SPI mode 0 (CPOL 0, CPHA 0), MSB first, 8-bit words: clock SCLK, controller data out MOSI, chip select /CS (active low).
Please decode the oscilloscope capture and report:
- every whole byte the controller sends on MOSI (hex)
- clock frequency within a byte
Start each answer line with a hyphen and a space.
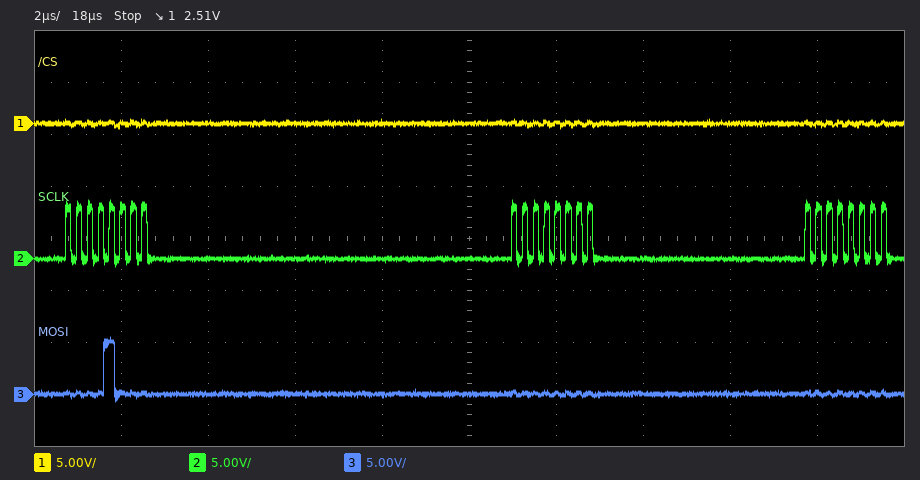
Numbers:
- 08 00 00
- 4 MHz
